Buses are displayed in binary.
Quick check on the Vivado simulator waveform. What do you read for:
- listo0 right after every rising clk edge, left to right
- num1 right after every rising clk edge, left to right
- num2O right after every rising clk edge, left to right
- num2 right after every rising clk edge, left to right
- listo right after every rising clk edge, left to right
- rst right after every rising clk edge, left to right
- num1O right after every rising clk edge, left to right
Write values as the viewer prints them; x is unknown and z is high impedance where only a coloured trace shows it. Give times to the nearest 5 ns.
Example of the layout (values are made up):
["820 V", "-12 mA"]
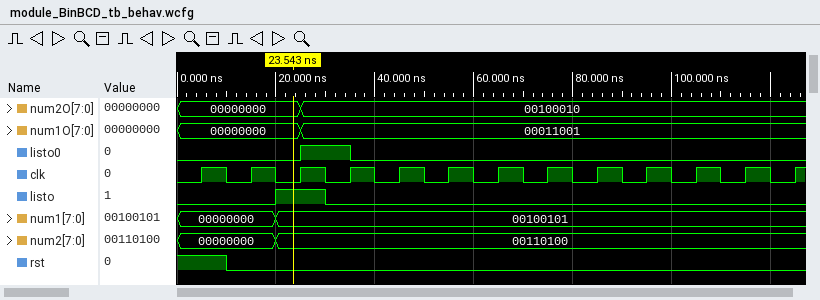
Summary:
["0 0 1 0 0 0 0 0 0 0 0 0 0", "00000000, 00000000, 00100101, 00100101, 00100101, 00100101, 00100101, 00100101, 00100101, 00100101, 00100101, 00100101, 00100101", "00000000, 00000000, 00100010, 00100010, 00100010, 00100010, 00100010, 00100010, 00100010, 00100010, 00100010, 00100010, 00100010", "00000000, 00000000, 00110100, 00110100, 00110100, 00110100, 00110100, 00110100, 00110100, 00110100, 00110100, 00110100, 00110100", "0 0 1 0 0 0 0 0 0 0 0 0 0", "1 0 0 0 0 0 0 0 0 0 0 0 0", "00000000, 00000000, 00011001, 00011001, 00011001, 00011001, 00011001, 00011001, 00011001, 00011001, 00011001, 00011001, 00011001"]
